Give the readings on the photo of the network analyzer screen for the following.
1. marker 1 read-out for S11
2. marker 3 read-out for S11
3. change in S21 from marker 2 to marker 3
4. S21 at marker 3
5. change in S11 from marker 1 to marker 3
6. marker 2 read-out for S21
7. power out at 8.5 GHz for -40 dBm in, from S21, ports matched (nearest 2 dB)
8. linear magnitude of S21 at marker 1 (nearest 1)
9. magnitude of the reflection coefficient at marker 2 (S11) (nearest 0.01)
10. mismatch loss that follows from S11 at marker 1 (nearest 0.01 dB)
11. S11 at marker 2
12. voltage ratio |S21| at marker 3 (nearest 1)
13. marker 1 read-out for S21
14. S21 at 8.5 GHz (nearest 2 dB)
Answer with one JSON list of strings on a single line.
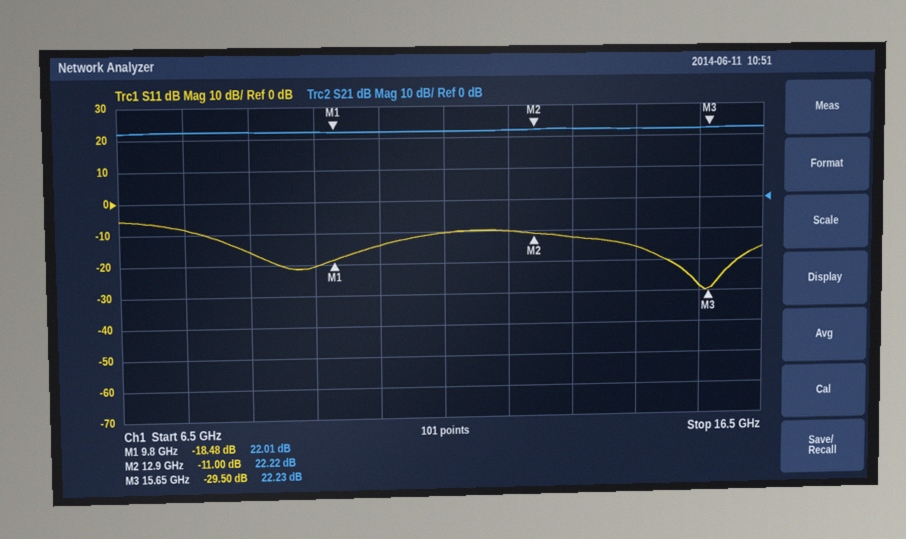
["-18.48 dB", "-29.50 dB", "0.01 dB", "22.23 dB", "-11.02 dB", "22.22 dB", "-18 dBm", "13", "0.28", "0.06 dB", "-11.00 dB", "13", "22.01 dB", "22 dB"]
